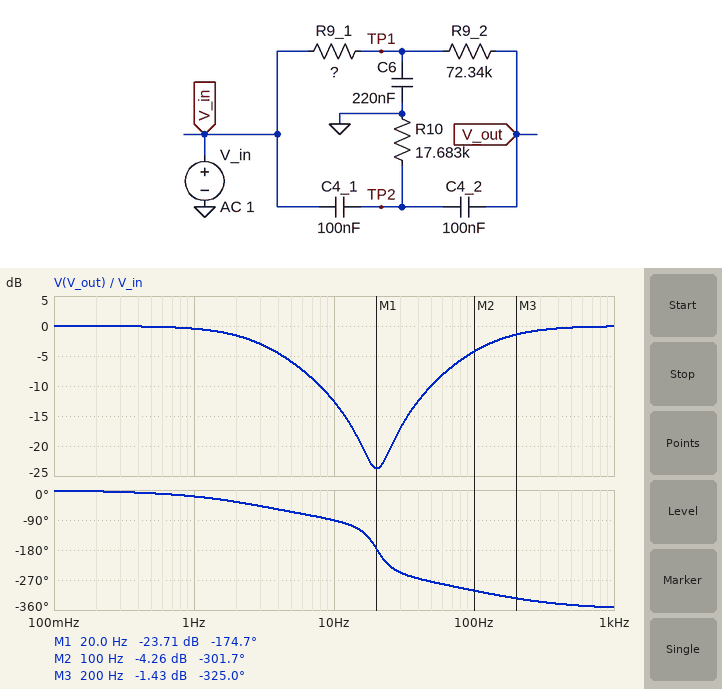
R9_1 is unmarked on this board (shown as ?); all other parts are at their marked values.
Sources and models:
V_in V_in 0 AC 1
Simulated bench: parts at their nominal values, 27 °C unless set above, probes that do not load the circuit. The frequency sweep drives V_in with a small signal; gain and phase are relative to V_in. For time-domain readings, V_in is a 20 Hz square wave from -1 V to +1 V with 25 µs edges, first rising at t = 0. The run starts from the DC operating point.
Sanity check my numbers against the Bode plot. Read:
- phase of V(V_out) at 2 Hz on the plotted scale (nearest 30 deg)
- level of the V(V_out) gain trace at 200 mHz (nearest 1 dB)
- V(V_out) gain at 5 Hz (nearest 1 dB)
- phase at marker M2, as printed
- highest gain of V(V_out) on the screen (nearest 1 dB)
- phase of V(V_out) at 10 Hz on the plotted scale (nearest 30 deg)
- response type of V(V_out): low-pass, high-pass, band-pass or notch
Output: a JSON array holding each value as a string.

["-30 deg", "0 dB", "-6 dB", "-301.7 deg", "0 dB", "-90 deg", "notch"]
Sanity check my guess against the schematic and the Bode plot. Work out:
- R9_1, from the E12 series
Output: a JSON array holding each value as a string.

["150 kΩ"]
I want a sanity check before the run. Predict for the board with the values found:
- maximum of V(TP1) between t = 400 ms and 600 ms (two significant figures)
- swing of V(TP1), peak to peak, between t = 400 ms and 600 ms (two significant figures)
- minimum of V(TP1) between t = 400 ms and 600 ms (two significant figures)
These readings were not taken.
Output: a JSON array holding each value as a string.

["290 mV", "570 mV", "-290 mV"]
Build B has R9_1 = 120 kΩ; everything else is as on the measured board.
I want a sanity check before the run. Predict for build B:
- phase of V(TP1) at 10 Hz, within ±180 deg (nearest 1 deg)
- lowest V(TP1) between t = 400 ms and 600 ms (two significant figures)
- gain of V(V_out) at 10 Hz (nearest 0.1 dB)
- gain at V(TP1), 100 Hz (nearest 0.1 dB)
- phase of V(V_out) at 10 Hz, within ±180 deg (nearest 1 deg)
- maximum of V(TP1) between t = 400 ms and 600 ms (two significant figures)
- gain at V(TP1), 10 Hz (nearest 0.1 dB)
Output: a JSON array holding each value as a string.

["-57 deg", "-350 mV", "-10.7 dB", "-19.6 dB", "-86 deg", "350 mV", "-8.8 dB"]
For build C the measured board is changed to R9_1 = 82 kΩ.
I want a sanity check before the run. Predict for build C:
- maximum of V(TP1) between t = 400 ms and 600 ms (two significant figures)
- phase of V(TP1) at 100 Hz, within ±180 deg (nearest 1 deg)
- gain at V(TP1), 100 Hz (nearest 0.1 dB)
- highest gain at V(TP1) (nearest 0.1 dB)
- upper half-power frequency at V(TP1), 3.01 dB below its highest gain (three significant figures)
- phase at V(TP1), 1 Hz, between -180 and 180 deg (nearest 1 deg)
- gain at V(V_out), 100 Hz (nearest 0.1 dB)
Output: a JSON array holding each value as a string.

["470 mV", "-56 deg", "-17.9 dB", "0 dB", "5.49 Hz", "-9 deg", "-4.4 dB"]
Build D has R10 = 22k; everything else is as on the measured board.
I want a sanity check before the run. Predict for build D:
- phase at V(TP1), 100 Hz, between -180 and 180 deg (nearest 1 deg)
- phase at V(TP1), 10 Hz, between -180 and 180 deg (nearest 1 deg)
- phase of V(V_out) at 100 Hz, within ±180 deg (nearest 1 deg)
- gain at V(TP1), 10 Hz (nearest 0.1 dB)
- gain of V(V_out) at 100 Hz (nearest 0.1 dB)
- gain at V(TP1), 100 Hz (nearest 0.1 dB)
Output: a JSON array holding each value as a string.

["-50 deg", "-59 deg", "53 deg", "-10.6 dB", "-3.5 dB", "-19.8 dB"]
